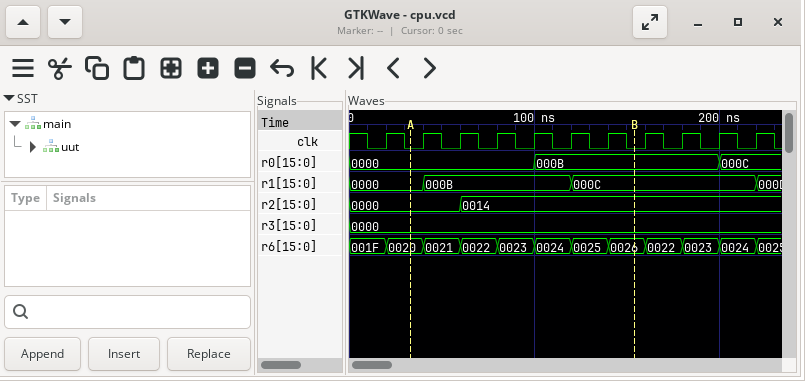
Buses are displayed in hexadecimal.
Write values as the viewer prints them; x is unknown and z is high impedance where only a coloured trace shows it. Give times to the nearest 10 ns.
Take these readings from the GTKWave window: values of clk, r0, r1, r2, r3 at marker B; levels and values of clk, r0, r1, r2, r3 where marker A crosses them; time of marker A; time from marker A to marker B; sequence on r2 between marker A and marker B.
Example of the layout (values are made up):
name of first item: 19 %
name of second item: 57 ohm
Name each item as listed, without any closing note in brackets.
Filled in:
values of clk, r0, r1, r2, r3 at marker B: clk=0, r0=000B, r1=000C, r2=0014, r3=0000
levels and values of clk, r0, r1, r2, r3 where marker A crosses them: clk=0, r0=0000, r1=0000, r2=0000, r3=0000
time of marker A: 30 ns
time from marker A to marker B: 120 ns
sequence on r2 between marker A and marker B: 0000, 0014
